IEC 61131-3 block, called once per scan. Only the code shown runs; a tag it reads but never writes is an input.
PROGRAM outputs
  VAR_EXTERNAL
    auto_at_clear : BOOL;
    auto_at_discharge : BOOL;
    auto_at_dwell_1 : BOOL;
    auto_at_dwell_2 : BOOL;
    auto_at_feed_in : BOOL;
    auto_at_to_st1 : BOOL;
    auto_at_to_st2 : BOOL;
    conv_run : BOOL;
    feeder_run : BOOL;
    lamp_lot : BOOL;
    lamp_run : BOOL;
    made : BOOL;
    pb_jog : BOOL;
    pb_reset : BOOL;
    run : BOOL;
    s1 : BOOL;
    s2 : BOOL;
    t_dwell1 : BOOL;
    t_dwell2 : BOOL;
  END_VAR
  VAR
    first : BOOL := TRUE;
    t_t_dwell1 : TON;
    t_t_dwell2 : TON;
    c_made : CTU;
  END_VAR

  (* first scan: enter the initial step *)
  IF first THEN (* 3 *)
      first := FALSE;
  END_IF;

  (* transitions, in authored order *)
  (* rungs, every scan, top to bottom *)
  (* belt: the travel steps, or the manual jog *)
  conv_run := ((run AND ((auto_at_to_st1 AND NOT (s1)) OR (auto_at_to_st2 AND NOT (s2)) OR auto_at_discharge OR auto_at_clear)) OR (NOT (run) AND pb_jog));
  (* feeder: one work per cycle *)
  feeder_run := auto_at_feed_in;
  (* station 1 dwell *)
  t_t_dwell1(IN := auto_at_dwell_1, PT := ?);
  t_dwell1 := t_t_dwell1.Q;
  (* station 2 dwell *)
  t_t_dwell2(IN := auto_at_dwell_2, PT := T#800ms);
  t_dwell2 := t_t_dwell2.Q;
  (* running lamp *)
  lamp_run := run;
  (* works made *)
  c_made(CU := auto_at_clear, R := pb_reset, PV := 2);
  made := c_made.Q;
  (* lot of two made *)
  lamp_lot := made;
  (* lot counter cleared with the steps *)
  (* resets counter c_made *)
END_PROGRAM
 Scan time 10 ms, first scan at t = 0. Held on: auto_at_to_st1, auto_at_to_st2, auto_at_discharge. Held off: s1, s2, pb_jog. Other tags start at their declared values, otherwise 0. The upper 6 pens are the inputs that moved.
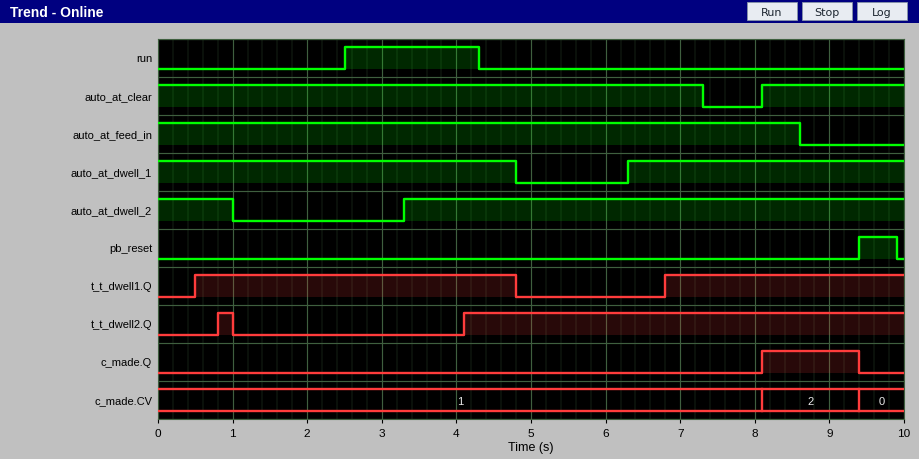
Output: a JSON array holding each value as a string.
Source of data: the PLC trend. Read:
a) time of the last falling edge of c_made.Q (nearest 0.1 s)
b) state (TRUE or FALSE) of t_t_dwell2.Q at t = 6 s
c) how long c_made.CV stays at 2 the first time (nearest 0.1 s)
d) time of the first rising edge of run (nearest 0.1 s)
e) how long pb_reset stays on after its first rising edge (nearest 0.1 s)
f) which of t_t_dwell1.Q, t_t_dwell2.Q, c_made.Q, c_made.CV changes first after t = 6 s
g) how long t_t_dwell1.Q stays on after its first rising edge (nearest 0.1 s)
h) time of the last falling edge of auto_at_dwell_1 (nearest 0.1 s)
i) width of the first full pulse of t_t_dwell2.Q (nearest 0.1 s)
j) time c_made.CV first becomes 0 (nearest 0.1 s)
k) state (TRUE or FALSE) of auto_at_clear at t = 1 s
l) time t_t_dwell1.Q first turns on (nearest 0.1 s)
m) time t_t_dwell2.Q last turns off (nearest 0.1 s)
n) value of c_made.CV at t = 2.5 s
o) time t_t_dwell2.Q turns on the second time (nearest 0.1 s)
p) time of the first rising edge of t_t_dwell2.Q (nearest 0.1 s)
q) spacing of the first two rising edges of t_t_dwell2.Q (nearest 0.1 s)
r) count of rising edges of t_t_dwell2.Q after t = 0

["9.4 s", "TRUE", "1.3 s", "2.5 s", "0.5 s", "t_t_dwell1.Q", "4.3 s", "4.8 s", "0.2 s", "9.4 s", "TRUE", "0.5 s", "1.0 s", "1", "4.1 s", "0.8 s", "3.3 s", "2"]
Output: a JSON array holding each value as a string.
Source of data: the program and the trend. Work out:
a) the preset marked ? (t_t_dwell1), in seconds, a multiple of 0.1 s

["0.5 s"]
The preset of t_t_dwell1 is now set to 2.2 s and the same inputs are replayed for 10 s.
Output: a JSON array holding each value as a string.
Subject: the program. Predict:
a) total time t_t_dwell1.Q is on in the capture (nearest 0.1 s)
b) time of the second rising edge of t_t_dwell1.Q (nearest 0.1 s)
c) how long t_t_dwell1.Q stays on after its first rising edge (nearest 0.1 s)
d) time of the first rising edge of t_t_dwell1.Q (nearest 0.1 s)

["4.1 s", "8.5 s", "2.6 s", "2.2 s"]
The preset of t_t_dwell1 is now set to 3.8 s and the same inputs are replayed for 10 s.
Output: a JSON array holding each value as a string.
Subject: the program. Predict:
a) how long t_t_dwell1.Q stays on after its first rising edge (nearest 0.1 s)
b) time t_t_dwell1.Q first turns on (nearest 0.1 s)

["1.0 s", "3.8 s"]
